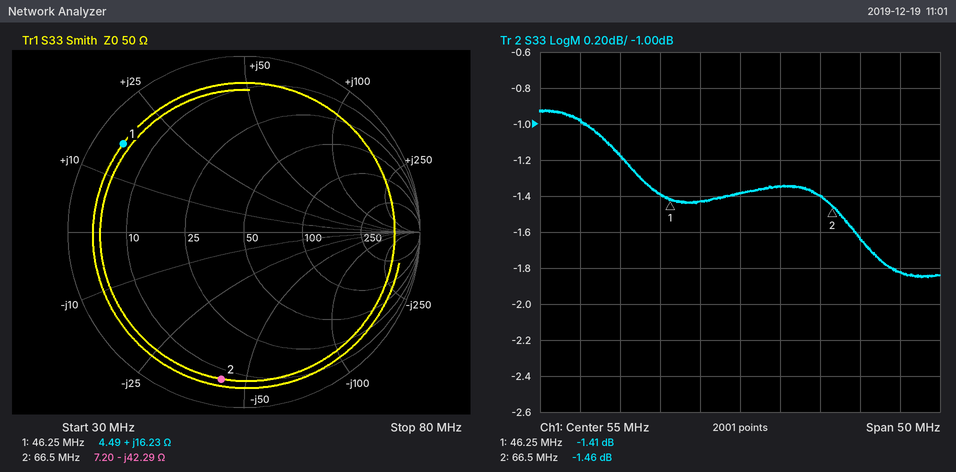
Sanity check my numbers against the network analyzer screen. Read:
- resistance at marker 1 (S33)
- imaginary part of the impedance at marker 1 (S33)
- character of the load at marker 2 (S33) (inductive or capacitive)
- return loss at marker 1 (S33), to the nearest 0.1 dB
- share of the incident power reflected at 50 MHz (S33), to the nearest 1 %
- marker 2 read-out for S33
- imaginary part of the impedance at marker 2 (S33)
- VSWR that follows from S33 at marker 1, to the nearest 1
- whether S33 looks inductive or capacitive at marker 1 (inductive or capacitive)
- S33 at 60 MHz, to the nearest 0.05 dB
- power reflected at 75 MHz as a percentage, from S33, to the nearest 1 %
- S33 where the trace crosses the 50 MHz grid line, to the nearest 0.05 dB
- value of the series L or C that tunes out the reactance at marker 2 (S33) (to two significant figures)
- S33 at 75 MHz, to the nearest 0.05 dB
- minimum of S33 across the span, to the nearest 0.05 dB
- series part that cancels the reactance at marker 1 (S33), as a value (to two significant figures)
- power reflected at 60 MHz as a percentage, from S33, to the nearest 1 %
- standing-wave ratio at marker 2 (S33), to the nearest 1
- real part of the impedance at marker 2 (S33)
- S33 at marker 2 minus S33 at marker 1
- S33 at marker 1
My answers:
4.49 Ω
+16.23 Ω
capacitive
1.4 dB
72 %
-1.46 dB
-42.29 Ω
12
inductive
-1.35 dB
66 %
-1.45 dB
100 nH
-1.80 dB
-1.85 dB
210 pF
73 %
12
7.20 Ω
-0.05 dB
-1.41 dB
